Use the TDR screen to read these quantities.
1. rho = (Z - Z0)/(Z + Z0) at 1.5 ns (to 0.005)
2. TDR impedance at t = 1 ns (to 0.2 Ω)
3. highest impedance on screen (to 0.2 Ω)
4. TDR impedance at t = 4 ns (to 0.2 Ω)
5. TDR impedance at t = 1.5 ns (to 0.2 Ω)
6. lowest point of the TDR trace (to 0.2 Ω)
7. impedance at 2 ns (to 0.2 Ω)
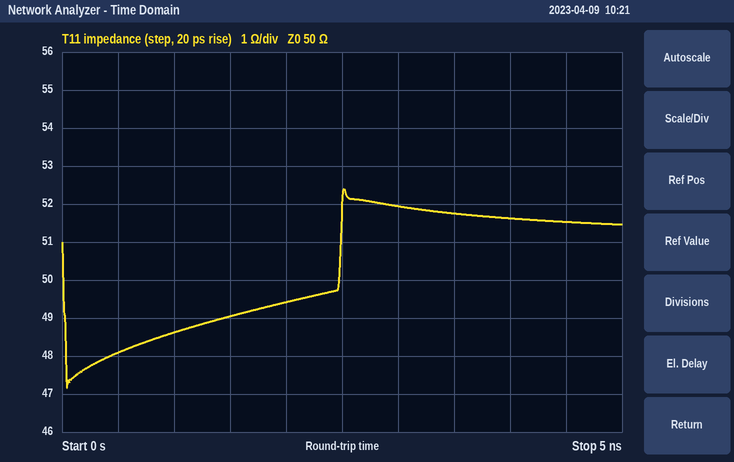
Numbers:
-0.010
48.6 Ω
52.4 Ω
51.6 Ω
49.0 Ω
47.2 Ω
49.4 Ω
